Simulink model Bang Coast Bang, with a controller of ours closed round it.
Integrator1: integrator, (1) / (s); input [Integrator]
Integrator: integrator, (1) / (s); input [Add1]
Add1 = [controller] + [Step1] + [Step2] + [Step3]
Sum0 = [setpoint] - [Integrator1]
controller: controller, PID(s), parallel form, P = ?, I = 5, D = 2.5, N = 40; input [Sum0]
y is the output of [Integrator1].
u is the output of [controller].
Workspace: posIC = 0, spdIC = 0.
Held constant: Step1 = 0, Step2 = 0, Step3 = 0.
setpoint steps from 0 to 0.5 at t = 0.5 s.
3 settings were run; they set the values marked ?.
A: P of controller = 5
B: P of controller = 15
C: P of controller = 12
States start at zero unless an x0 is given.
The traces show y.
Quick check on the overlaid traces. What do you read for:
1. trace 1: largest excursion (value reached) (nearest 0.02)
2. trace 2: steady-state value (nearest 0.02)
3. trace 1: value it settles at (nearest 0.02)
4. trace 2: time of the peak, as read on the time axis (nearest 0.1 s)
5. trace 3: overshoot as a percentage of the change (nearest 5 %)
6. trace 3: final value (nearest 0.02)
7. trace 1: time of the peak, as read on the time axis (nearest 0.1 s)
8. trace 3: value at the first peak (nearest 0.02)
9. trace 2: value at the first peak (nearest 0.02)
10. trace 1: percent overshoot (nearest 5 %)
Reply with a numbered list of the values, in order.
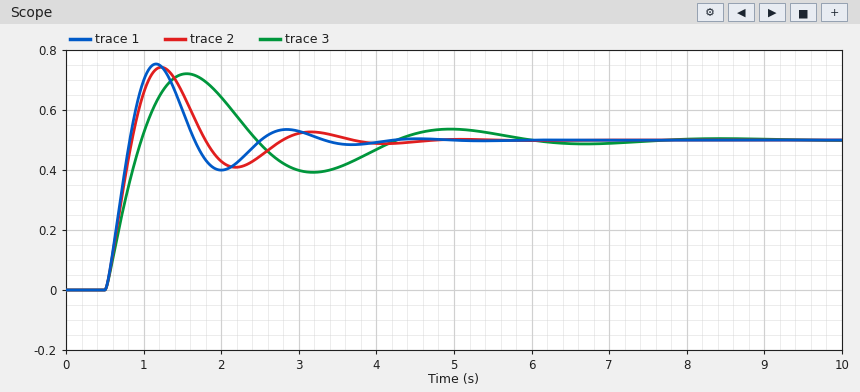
1. 0.76
2. 0.50
3. 0.50
4. 1.2 s
5. 45 %
6. 0.50
7. 1.2 s
8. 0.72
9. 0.74
10. 50 %
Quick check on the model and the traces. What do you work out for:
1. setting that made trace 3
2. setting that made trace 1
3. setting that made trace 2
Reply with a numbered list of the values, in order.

1. A
2. B
3. C
